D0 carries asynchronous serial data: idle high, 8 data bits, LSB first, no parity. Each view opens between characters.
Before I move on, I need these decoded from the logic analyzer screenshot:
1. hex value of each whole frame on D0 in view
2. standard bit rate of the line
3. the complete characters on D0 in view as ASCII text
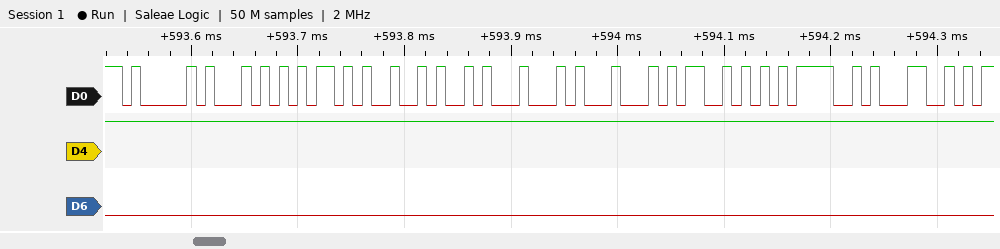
41, 54, 2B, 4A, 44, 44, 53, 3D, 31
115200 baud
"AT+JDDS=1"
